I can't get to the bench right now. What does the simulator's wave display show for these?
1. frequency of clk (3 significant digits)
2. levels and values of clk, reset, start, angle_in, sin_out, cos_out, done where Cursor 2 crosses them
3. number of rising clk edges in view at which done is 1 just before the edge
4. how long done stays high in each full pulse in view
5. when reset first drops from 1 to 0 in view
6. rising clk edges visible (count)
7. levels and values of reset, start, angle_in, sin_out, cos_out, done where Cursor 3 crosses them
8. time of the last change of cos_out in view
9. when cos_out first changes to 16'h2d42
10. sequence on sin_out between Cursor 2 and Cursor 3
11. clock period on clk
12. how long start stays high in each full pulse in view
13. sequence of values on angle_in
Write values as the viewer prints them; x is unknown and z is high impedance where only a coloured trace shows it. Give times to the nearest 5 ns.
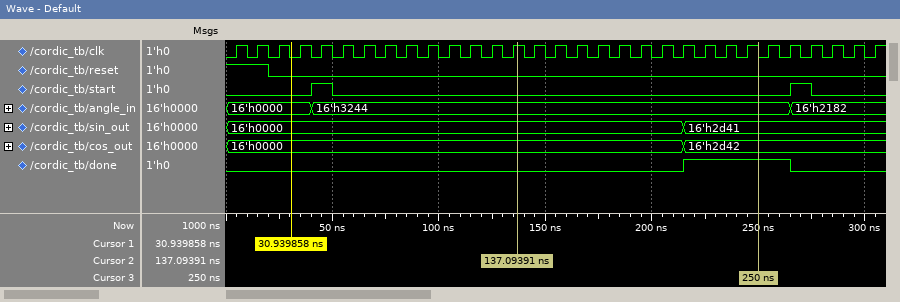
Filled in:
100 MHz
clk=1, reset=0, start=0, angle_in=16'h3244, sin_out=16'h0000, cos_out=16'h0000, done=0
5
50 ns
20 ns
31
reset=0, start=0, angle_in=16'h3244, sin_out=16'h2d41, cos_out=16'h2d42, done=1
215 ns
215 ns
16'h0000, 16'h2d41
10 ns
10 ns, 10 ns
16'h0000, 16'h3244, 16'h2182
